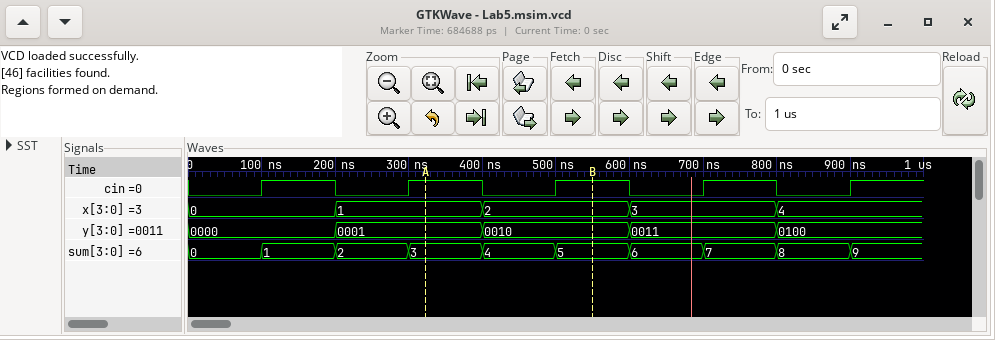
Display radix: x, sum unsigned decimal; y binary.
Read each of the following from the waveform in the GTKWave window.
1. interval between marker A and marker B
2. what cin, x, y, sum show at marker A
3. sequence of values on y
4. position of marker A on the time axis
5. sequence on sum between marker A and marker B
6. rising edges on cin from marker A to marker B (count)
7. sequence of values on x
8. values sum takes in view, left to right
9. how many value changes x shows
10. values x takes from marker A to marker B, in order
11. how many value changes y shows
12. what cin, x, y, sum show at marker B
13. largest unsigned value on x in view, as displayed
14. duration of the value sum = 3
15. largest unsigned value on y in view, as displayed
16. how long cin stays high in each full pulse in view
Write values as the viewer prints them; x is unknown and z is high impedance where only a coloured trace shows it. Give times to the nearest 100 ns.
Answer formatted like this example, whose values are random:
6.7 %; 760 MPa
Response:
200 ns; cin=1, x=1, y=0001, sum=3; 0000, 0001, 0010, 0011, 0100; 300 ns; 3, 4, 5; 1; 0, 1, 2, 3, 4; 0, 1, 2, 3, 4, 5, 6, 7, 8, 9; 4; 1, 2; 4; cin=1, x=2, y=0010, sum=5; 4; 100 ns; 0100; 100 ns, 100 ns, 100 ns, 100 ns
